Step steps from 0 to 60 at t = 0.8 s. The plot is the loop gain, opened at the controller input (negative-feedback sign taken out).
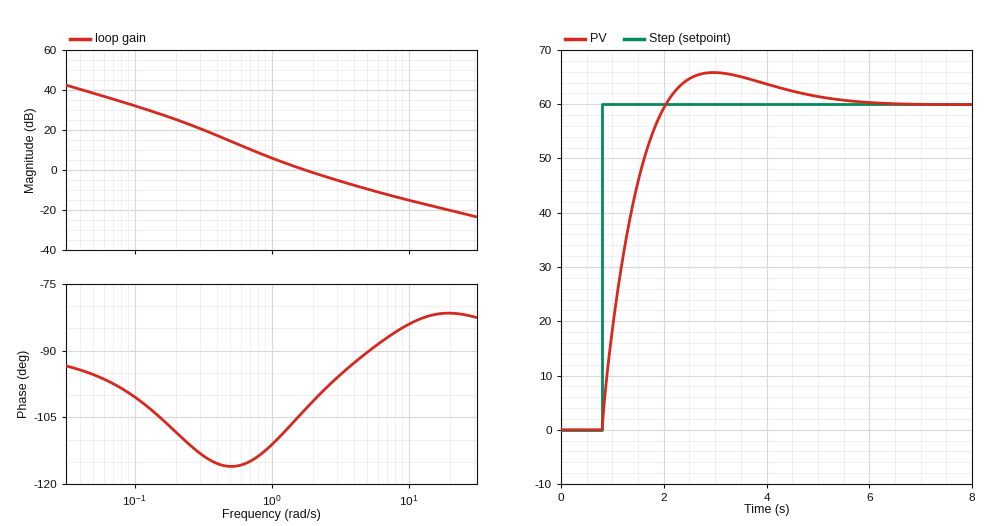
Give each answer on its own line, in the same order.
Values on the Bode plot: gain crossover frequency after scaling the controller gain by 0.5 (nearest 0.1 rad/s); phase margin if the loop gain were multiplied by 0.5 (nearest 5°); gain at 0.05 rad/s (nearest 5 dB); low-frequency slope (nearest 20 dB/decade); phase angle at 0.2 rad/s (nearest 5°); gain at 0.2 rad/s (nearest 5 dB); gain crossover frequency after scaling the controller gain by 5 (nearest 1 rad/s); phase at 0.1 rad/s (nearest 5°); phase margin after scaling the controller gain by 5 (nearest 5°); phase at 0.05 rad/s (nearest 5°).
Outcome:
1.0 rad/s
70°
40 dB
-20 dB/decade
-110°
25 dB
9 rad/s
-100°
95°
-95°
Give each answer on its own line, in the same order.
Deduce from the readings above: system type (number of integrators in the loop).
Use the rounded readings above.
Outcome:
1
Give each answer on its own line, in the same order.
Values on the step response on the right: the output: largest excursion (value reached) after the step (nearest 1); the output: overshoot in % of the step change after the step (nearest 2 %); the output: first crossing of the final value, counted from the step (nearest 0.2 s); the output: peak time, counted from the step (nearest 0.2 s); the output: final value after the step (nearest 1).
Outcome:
66
10 %
1.2 s
2.2 s
60
